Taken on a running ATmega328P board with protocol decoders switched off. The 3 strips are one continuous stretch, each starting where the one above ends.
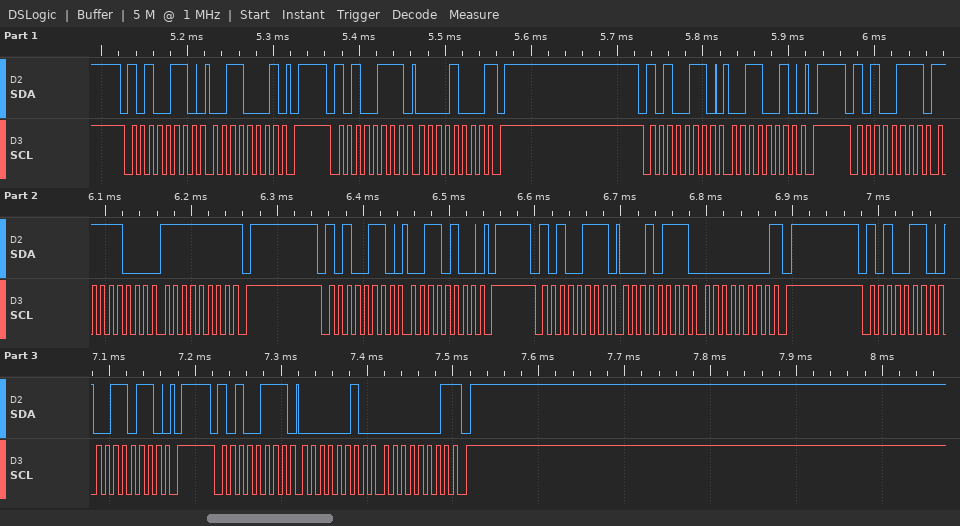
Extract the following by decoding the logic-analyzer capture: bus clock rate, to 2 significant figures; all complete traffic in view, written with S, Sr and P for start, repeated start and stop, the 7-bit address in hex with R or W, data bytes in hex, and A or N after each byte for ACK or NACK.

100 kHz
S 53W A 31 A P S 53R A 08 N P S 53W A 32 A P S 53R A F8 A FF N P S 53W A 34 A P S 53R A 17 A 00 N P S 53W A 36 A P S 53R A 02 A 01 N P
